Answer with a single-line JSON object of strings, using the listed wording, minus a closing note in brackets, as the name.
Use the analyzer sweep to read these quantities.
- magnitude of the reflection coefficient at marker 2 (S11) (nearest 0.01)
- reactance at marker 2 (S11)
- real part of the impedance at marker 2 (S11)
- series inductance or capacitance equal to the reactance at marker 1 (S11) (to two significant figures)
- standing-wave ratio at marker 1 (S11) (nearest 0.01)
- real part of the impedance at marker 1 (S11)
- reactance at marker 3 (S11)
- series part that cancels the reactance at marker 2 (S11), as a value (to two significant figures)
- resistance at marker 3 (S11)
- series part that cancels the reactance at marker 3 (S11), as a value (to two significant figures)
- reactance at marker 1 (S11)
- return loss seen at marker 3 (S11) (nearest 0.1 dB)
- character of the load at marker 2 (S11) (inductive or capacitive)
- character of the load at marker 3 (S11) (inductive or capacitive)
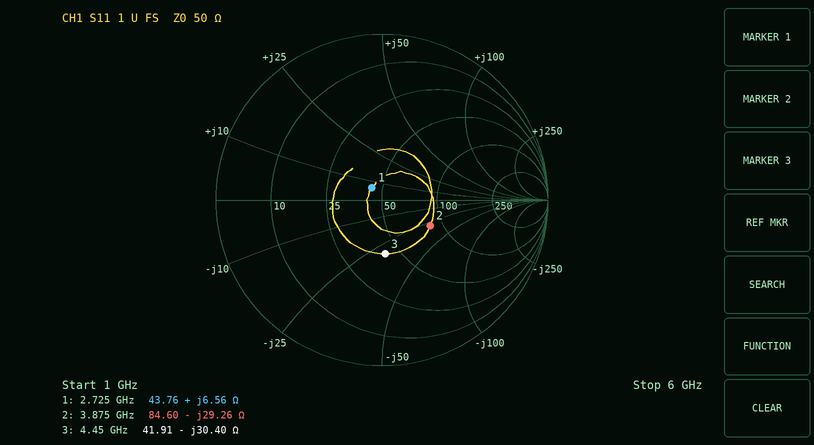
{"magnitude of the reflection coefficient at marker 2 (S11)": "0.33", "reactance at marker 2": "-29.26 Ω", "real part of the impedance at marker 2": "84.60 Ω", "series inductance or capacitance equal to the reactance at marker 1 (S11)": "380 pH", "standing-wave ratio at marker 1 (S11)": "1.21", "real part of the impedance at marker 1": "43.76 Ω", "reactance at marker 3": "-30.40 Ω", "series part that cancels the reactance at marker 2 (S11), as a value": "1.2 nH", "resistance at marker 3": "41.91 Ω", "series part that cancels the reactance at marker 3 (S11), as a value": "1.1 nH", "reactance at marker 1": "+6.56 Ω", "return loss seen at marker 3 (S11)": "9.8 dB", "character of the load at marker 2 (S11)": "capacitive", "character of the load at marker 3 (S11)": "capacitive"}
